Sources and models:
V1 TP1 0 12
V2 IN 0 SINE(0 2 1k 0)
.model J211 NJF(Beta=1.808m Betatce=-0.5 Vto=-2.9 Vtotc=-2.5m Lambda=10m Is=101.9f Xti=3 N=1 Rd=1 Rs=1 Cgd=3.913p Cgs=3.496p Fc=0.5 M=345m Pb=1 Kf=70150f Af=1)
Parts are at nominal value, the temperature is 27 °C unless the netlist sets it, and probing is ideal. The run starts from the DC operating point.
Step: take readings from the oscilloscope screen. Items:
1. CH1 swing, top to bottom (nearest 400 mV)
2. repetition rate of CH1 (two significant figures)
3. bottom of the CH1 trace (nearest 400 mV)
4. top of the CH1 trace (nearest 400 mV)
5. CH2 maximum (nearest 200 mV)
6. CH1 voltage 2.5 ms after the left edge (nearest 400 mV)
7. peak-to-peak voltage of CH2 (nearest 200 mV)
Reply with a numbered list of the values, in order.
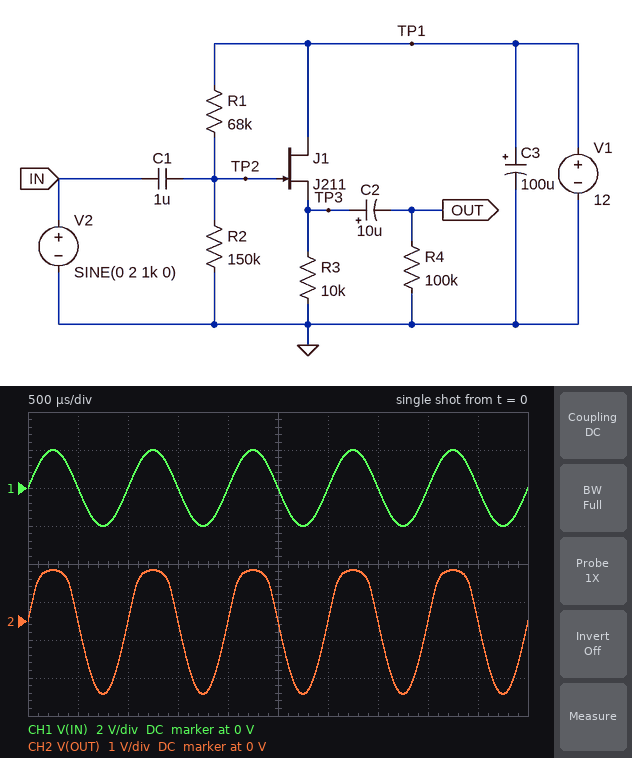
1. 4.0 V
2. 1.0 kHz
3. -2.0 V
4. 2.0 V
5. 1.4 V
6. 0 V
7. 3.2 V
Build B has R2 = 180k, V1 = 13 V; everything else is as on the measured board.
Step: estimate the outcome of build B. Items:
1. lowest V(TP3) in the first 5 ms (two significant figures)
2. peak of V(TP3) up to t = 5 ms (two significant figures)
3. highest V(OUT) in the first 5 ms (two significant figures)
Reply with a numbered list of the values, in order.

1. 9.6 V
2. 13 V
3. 1.2 V
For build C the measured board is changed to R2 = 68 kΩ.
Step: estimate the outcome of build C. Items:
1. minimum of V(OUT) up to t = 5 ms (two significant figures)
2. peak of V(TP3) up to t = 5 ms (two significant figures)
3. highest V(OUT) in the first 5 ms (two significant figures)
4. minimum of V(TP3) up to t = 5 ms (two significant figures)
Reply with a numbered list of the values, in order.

1. -1.9 V
2. 10 V
3. 1.9 V
4. 6.3 V
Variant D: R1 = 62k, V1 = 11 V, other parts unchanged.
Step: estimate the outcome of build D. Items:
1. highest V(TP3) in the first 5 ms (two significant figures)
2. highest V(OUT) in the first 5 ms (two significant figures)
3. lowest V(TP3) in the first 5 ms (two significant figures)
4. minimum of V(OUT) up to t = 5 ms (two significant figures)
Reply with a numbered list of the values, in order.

1. 11 V
2. 880 mV
3. 8.0 V
4. -1.9 V
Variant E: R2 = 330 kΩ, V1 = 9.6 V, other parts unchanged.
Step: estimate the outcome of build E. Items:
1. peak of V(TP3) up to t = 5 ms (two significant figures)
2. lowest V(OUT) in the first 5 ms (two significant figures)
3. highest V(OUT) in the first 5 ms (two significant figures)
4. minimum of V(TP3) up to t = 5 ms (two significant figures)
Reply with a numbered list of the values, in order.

1. 9.5 V
2. -1.2 V
3. 110 mV
4. 8.2 V
